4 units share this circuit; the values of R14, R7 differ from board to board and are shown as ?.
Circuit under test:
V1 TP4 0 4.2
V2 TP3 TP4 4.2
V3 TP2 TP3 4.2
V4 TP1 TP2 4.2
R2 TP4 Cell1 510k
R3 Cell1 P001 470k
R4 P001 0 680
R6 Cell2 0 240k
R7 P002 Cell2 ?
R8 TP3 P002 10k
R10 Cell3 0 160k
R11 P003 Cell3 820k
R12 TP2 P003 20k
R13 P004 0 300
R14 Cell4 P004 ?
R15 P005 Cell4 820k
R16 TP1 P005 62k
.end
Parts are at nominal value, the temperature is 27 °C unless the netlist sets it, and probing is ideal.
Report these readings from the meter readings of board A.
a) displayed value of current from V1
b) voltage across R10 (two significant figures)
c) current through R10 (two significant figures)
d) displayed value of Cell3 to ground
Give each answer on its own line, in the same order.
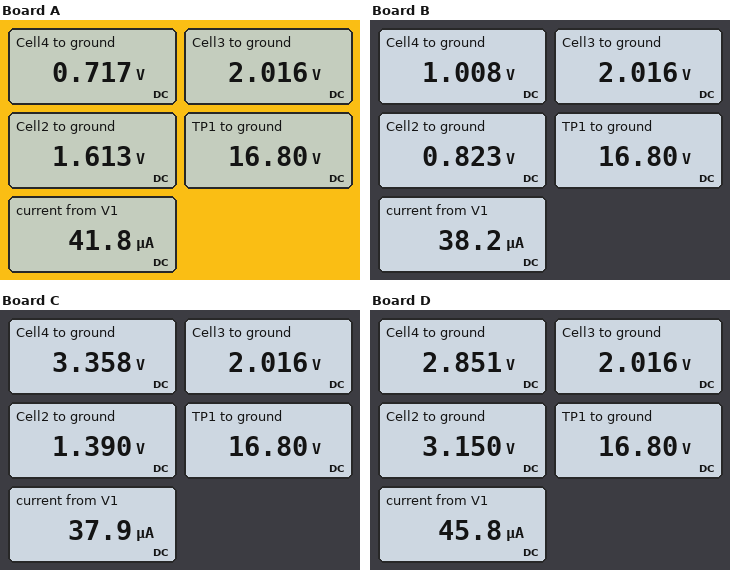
41.8 µA
2.0 V
13 µA
2.016 V
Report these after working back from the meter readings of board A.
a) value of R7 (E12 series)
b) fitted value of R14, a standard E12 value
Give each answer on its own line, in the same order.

1 MΩ
39 kΩ
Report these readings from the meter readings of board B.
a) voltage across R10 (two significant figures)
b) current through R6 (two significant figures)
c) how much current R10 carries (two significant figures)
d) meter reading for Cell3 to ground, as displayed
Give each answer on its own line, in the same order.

2.0 V
3.4 µA
13 µA
2.016 V
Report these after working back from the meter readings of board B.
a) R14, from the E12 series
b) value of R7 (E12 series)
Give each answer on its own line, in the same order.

56 kΩ
2.2 MΩ
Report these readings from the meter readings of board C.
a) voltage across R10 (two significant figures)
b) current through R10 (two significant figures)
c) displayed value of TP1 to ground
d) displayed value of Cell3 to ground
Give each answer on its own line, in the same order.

2.0 V
13 µA
16.80 V
2.016 V
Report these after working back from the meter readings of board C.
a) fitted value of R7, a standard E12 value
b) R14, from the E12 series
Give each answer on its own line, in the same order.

1.2 MΩ
220 kΩ
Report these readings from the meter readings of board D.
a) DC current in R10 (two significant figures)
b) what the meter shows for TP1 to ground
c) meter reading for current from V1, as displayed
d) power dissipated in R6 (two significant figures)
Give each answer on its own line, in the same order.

13 µA
16.80 V
45.8 µA
41 µW
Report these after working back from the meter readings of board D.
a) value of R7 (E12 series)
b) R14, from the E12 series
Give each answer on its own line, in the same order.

390 kΩ
180 kΩ
